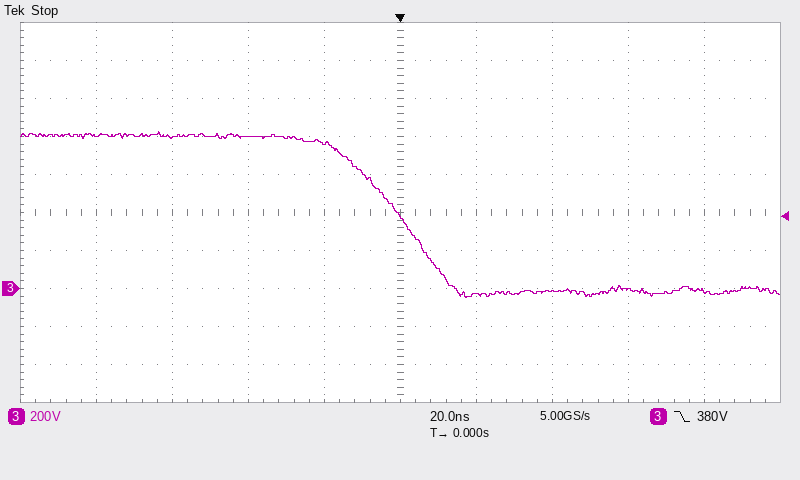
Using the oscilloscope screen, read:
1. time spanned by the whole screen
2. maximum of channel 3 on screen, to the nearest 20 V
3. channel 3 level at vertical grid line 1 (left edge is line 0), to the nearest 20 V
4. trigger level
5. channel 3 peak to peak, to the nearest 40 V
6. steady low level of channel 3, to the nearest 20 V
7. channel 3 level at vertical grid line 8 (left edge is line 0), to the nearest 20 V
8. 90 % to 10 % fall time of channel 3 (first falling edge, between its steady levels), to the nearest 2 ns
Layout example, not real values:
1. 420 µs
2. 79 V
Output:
1. 200 ns
2. 820 V
3. 800 V
4. 380 V
5. 880 V
6. -20 V
7. 0 V
8. 28 ns
